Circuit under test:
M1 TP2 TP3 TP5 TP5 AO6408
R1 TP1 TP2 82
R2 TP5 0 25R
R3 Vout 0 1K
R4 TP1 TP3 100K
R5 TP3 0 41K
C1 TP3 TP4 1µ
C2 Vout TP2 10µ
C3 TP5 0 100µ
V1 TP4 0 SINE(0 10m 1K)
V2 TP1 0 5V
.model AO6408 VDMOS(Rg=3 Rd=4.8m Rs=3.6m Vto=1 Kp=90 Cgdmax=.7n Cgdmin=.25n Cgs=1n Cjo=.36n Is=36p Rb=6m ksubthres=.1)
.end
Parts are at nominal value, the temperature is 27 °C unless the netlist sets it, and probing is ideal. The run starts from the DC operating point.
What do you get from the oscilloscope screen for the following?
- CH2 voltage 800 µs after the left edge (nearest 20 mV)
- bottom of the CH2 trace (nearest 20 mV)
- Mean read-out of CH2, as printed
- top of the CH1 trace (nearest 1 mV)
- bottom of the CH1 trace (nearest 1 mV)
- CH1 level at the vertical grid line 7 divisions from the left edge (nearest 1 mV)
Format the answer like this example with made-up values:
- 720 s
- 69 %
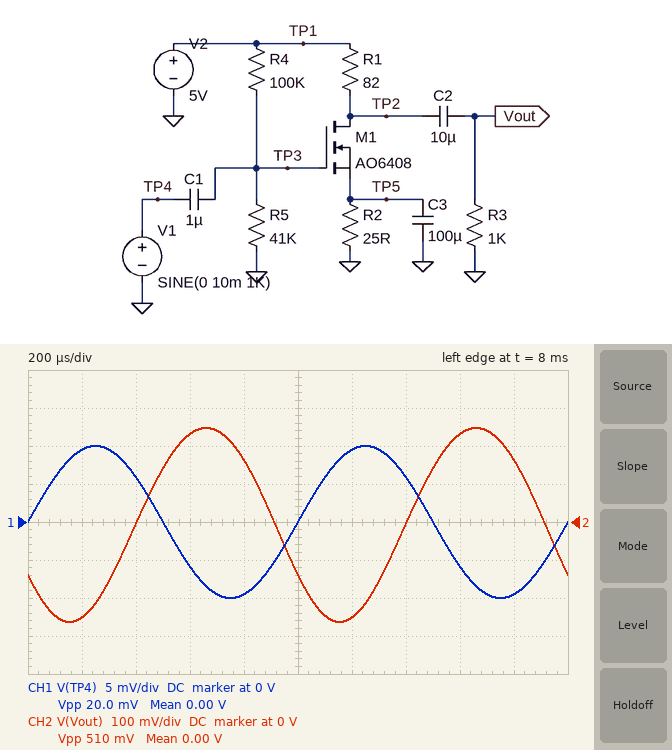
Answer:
- 160 mV
- -260 mV
- 0.00 V
- 10 mV
- -10 mV
- 6 mV
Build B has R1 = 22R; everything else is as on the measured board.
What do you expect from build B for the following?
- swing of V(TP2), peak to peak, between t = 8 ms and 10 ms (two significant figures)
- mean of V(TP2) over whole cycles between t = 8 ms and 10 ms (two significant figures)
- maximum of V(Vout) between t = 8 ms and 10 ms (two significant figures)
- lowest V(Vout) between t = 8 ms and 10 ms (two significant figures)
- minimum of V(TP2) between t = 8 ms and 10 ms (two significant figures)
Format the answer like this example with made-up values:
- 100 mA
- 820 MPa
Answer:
- 150 mV
- 4.5 V
- 71 mV
- -75 mV
- 4.4 V
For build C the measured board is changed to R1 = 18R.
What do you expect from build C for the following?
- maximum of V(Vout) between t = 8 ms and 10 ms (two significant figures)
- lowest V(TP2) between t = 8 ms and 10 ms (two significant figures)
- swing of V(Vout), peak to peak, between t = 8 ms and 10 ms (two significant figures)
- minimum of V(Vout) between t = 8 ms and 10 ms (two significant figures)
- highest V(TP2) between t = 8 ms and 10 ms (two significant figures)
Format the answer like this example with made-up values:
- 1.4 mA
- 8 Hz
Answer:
- 58 mV
- 4.5 V
- 120 mV
- -62 mV
- 4.6 V
